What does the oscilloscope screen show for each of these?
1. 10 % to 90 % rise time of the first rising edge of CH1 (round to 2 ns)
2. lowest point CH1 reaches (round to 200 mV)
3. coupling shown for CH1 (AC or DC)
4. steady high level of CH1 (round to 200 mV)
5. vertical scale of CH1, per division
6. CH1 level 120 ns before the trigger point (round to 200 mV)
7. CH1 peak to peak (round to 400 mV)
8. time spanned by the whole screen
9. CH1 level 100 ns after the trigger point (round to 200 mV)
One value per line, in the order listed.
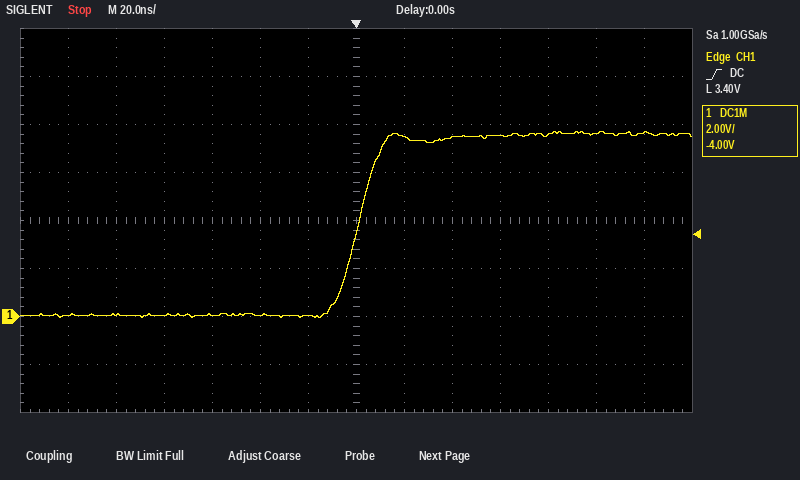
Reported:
18 ns
0.0 V
DC
7.6 V
2 V
0.0 V
7.6 V
280 ns
7.6 V
